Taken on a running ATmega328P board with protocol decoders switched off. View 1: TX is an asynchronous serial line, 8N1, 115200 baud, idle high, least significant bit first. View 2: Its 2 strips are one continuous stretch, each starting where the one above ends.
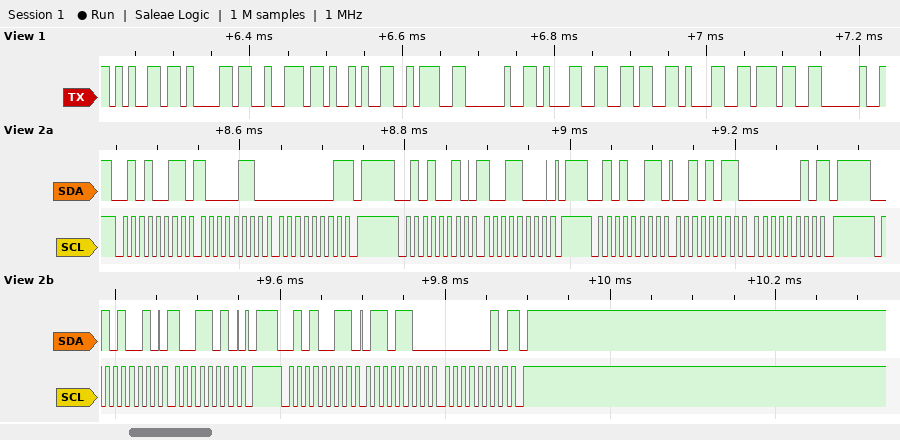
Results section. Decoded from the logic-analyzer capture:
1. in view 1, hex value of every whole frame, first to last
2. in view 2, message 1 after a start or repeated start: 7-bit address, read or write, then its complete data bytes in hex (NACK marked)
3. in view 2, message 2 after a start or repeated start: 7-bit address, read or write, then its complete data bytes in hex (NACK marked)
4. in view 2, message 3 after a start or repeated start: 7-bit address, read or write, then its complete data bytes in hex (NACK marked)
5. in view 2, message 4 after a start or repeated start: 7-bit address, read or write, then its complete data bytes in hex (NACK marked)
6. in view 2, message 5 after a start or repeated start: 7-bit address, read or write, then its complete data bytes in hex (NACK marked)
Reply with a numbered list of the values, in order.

1. 65 61 72 29 3A 20 31 36 31 37 20
2. 0x29 read: 86 01 NACK
3. 0x29 write: 98
4. 0x29 read: 2B 02 NACK
5. 0x29 write: 9A
6. 0x29 read: 6C 02 NACK
